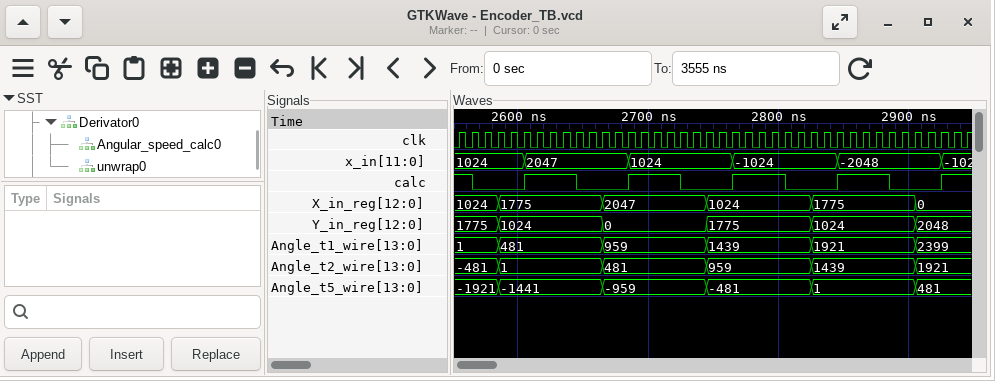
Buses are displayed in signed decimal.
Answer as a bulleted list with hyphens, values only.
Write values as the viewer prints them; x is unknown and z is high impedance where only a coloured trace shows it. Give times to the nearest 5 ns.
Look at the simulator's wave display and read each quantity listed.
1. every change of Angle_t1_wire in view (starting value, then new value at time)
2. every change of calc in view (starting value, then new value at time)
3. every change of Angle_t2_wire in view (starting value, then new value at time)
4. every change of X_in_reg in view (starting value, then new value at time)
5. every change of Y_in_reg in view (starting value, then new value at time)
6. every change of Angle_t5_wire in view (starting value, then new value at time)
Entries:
- 1, 481 at 2585 ns, 959 at 2665 ns, 1439 at 2745 ns, 1921 at 2825 ns, 2399 at 2905 ns
- 1, 0 at 2565 ns, 1 at 2605 ns, 0 at 2645 ns, 1 at 2685 ns, 0 at 2725 ns, 1 at 2765 ns, 0 at 2805 ns, 1 at 2845 ns, 0 at 2885 ns, 1 at 2925 ns
- -481, 1 at 2585 ns, 481 at 2665 ns, 959 at 2745 ns, 1439 at 2825 ns, 1921 at 2905 ns
- 1024, 1775 at 2585 ns, 2047 at 2665 ns, 1024 at 2745 ns, 1775 at 2825 ns, 0 at 2905 ns
- 1775, 1024 at 2585 ns, 0 at 2665 ns, 1775 at 2745 ns, 1024 at 2825 ns, 2048 at 2905 ns
- -1921, -1441 at 2585 ns, -959 at 2665 ns, -481 at 2745 ns, 1 at 2825 ns, 481 at 2905 ns
